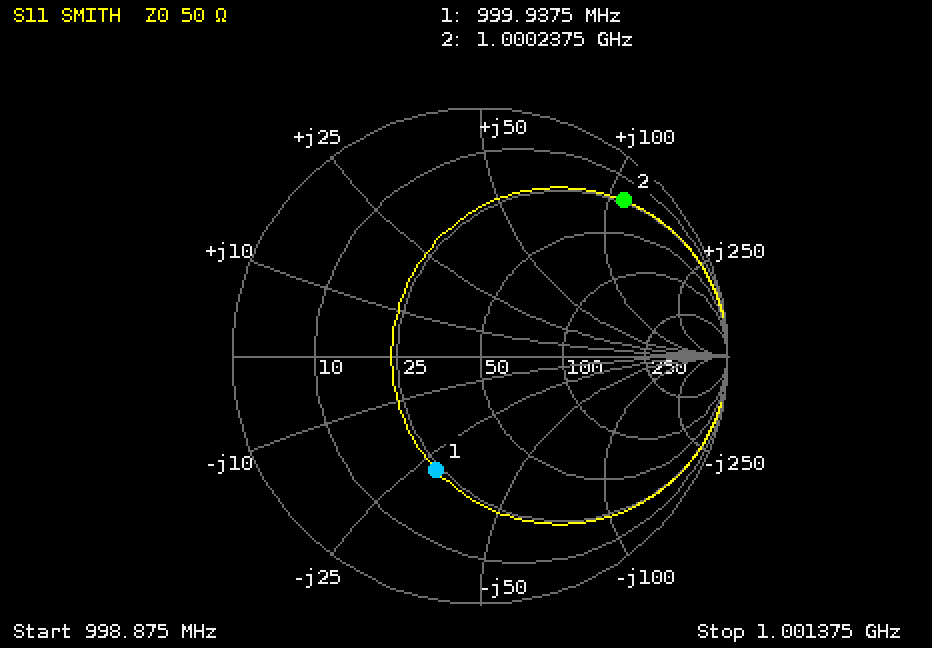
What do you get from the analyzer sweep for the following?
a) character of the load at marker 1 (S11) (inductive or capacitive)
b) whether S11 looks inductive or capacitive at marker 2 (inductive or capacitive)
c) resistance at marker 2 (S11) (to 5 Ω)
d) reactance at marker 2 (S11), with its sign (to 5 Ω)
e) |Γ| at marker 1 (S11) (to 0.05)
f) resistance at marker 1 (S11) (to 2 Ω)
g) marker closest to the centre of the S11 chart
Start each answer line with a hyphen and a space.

- capacitive
- inductive
- 25 Ω
- +110 Ω
- 0.50
- 24 Ω
- marker 1
